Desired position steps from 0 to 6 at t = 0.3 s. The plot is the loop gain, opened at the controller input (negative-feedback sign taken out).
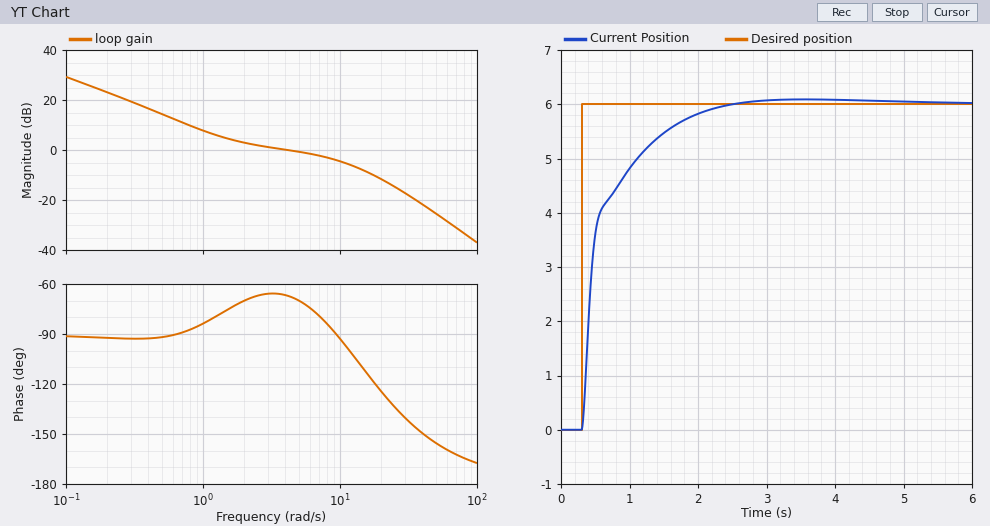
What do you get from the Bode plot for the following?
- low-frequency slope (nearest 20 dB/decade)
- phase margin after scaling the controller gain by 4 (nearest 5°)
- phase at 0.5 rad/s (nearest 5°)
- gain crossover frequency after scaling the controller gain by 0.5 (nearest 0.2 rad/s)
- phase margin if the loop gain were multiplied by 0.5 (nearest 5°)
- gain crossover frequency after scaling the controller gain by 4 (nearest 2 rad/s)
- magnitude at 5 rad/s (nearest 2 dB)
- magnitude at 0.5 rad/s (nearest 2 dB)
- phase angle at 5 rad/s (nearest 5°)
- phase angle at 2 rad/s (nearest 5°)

-20 dB/decade
55°
-90°
1.2 rad/s
100°
20 rad/s
0 dB
14 dB
-70°
-70°
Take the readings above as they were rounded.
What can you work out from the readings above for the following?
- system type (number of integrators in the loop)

1
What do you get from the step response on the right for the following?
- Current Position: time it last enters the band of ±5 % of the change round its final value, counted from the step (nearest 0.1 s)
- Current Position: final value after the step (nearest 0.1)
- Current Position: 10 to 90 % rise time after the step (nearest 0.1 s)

1.5 s
6.0
1.1 s
